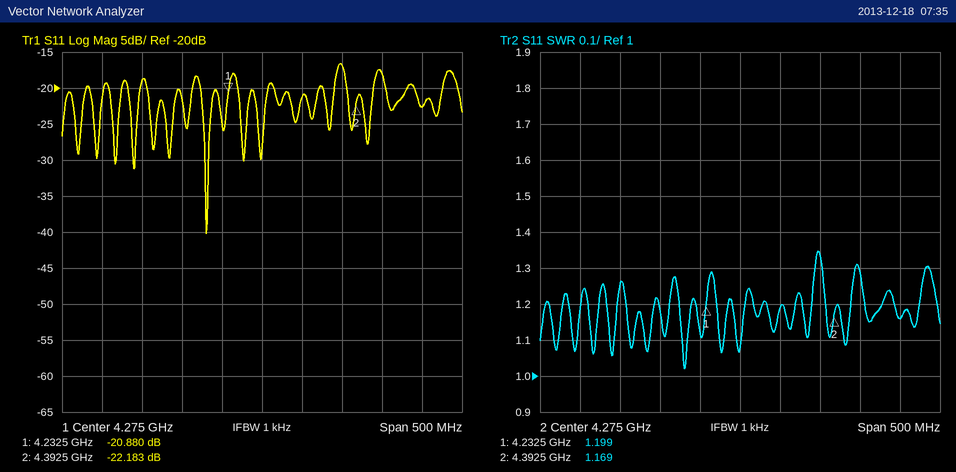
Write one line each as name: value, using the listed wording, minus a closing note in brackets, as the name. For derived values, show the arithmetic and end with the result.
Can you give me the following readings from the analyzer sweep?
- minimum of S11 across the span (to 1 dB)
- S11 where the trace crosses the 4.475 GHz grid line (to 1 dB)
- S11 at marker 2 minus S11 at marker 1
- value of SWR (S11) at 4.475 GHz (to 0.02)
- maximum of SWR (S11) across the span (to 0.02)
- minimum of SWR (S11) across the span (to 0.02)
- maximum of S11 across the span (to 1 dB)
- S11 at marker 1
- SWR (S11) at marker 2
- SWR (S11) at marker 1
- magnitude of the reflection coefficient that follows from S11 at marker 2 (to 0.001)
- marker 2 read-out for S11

minimum of S11 across the span: -40 dB
S11 where the trace crosses the 4.475 GHz grid line: -23 dB
S11 at marker 2 minus S11 at marker 1: -22.183 − (-20.88) = -1.303 dB
value of SWR (S11) at 4.475 GHz: 1.16
maximum of SWR (S11) across the span: 1.34
minimum of SWR (S11) across the span: 1.02
maximum of S11 across the span: -17 dB
S11 at marker 1: -20.880 dB
SWR (S11) at marker 2: 1.169
SWR (S11) at marker 1: 1.199
magnitude of the reflection coefficient that follows from S11 at marker 2: 10^(-22.183/20) ≈ 0.078
marker 2 read-out for S11: -22.183 dB
